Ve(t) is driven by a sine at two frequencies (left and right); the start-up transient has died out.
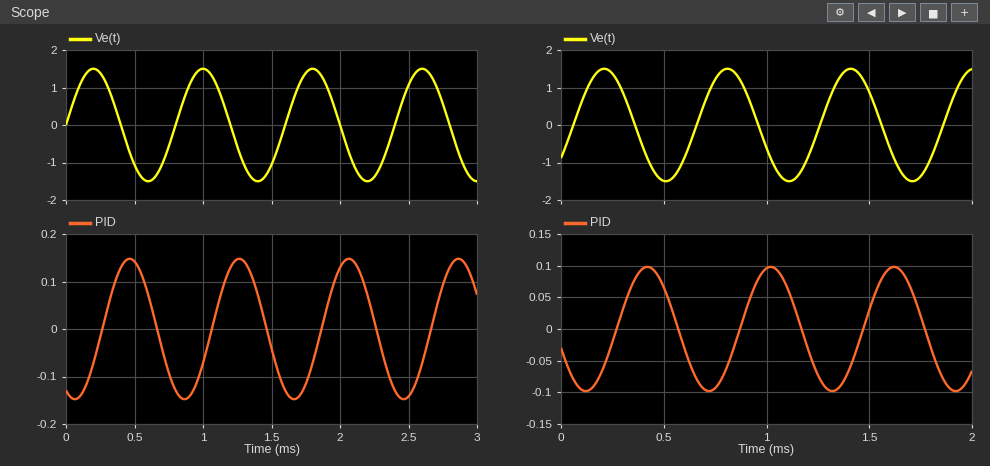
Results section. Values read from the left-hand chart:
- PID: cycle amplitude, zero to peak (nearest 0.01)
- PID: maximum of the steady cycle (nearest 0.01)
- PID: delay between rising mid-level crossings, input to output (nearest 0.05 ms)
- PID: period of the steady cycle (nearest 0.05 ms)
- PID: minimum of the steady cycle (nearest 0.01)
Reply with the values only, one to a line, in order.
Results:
0.15
0.15
0.25 ms
0.80 ms
-0.15
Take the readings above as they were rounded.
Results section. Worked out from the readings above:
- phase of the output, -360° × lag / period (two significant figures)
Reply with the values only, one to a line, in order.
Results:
-110°
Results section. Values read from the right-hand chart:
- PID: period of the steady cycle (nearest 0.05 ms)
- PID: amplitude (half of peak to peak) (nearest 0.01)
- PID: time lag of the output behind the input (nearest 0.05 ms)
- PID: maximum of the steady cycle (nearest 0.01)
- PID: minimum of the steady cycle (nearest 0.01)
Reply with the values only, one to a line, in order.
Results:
0.60 ms
0.10
0.20 ms
0.10
-0.10
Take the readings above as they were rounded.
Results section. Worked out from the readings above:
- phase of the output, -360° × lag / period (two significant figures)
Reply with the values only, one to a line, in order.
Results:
-120°
